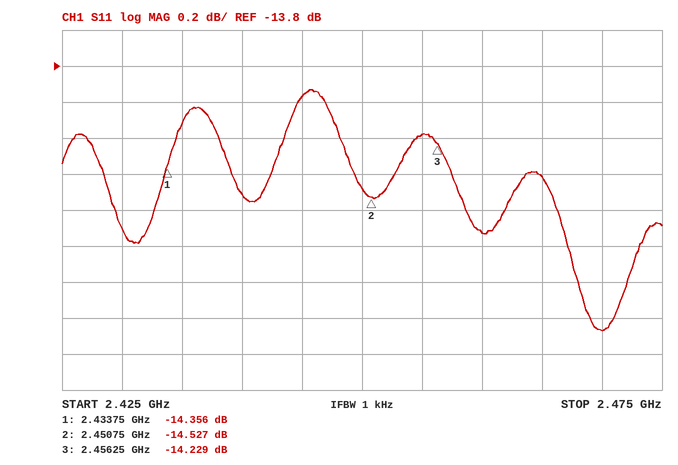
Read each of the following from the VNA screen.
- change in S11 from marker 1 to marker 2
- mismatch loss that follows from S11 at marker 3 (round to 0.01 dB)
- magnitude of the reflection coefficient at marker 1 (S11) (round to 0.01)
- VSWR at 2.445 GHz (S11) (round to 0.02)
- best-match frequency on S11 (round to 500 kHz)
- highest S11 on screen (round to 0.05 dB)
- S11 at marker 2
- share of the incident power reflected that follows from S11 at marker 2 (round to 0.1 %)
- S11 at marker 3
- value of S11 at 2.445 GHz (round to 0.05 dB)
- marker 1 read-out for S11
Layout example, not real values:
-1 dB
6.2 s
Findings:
-0.171 dB
0.17 dB
0.19
1.50
2.4700 GHz
-13.95 dB
-14.527 dB
3.5 %
-14.229 dB
-13.95 dB
-14.356 dB
